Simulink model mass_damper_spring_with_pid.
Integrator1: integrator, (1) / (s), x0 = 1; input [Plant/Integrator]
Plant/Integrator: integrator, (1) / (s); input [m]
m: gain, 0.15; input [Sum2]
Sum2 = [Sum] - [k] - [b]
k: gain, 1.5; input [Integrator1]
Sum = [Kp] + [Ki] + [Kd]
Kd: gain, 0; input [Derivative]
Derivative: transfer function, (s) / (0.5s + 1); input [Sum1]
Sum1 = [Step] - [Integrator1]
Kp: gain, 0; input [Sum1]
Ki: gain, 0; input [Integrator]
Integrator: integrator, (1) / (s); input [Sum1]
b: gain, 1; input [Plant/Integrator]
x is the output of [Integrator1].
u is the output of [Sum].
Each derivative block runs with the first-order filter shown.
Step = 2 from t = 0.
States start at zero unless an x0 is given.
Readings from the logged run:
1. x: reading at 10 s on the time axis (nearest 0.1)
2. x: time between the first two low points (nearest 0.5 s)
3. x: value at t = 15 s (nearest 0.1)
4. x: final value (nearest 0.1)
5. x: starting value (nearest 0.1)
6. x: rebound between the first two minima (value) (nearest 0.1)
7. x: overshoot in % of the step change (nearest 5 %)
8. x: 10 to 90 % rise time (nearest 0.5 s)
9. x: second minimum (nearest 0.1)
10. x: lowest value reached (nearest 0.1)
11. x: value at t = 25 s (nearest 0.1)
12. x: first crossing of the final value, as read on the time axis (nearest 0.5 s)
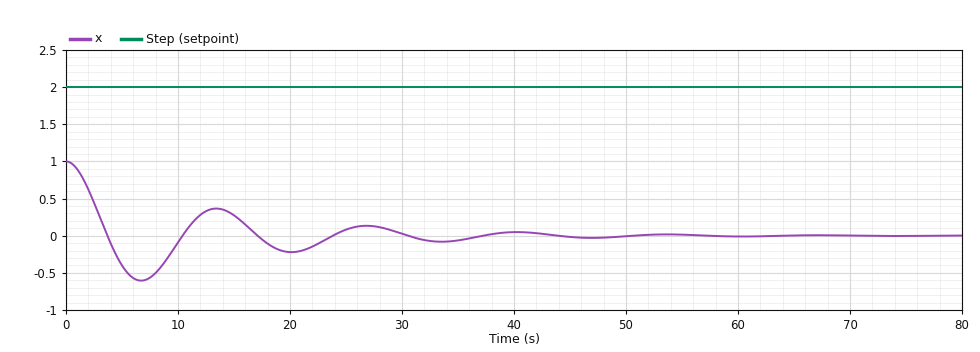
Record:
-0.1
13.5 s
0.3
0.0
1.0
0.4
60 %
2.5 s
-0.2
-0.6
0.1
3.5 s
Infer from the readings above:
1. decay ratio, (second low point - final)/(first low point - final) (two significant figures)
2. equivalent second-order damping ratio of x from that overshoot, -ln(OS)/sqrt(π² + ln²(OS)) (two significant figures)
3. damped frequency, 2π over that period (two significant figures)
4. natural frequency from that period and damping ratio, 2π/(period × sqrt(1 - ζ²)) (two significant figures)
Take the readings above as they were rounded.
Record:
0.33
0.16
0.47 rad/s
0.47 rad/s
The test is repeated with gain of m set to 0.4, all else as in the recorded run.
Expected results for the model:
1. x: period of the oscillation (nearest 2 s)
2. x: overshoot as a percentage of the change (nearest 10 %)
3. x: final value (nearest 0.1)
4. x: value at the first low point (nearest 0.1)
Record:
8 s
40 %
0.0
-0.4
